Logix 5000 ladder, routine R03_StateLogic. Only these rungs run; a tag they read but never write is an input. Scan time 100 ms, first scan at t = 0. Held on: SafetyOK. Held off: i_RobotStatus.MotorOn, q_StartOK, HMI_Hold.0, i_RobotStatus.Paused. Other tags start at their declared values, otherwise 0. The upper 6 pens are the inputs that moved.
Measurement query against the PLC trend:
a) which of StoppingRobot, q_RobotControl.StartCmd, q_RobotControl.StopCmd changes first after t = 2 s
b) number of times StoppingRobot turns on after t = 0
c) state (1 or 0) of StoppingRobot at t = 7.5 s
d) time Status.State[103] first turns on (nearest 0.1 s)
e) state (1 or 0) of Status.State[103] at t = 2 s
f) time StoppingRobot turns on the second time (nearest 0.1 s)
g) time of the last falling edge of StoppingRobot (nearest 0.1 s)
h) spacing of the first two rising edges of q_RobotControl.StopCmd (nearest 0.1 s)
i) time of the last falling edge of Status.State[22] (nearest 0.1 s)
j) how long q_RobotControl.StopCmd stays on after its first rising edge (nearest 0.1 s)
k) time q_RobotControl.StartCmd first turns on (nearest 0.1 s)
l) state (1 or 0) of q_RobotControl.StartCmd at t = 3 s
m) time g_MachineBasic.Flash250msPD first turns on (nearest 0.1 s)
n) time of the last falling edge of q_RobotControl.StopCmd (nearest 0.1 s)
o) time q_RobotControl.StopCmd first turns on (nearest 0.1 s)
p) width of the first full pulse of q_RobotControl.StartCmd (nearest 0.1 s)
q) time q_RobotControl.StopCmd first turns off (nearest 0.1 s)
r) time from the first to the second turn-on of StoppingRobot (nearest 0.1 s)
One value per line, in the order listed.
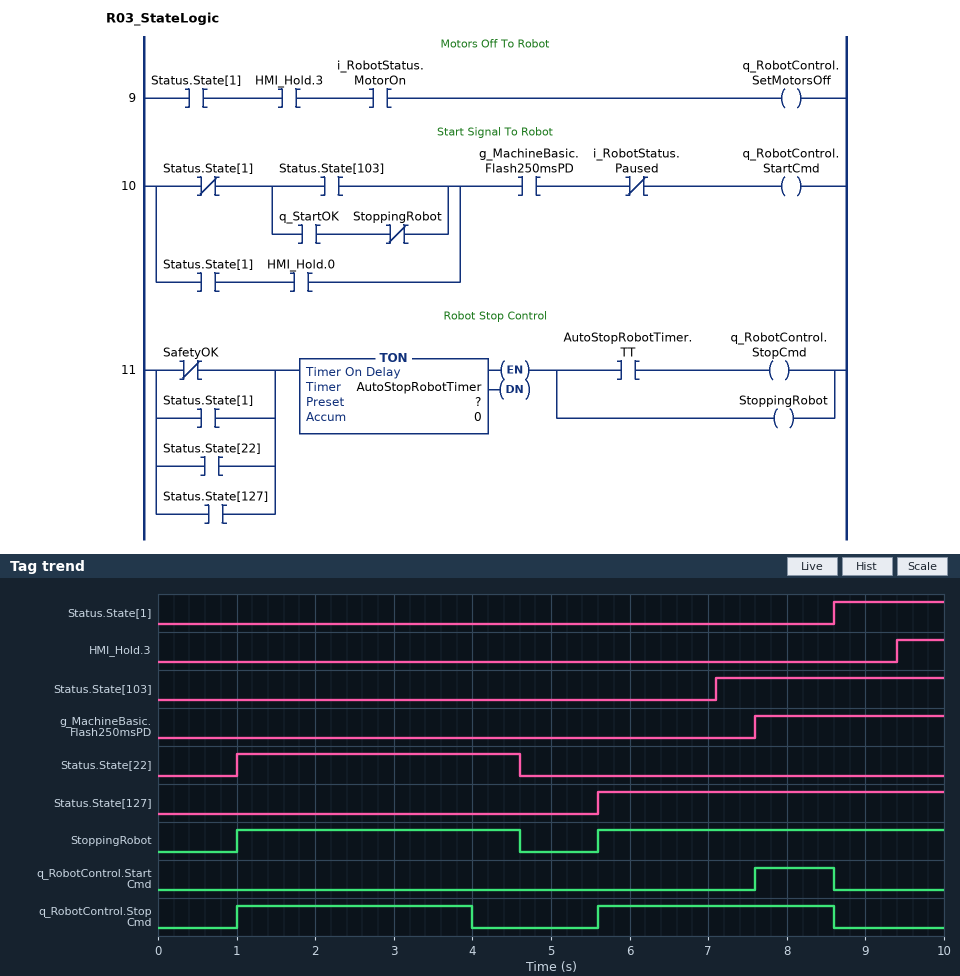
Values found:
q_RobotControl.StopCmd
2
1
7.1 s
0
5.6 s
4.6 s
4.6 s
4.6 s
3.0 s
7.6 s
0
7.6 s
8.6 s
1.0 s
1.0 s
4.0 s
4.6 s
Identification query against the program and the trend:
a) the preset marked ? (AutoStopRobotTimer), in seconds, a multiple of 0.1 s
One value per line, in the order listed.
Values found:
3.0 s
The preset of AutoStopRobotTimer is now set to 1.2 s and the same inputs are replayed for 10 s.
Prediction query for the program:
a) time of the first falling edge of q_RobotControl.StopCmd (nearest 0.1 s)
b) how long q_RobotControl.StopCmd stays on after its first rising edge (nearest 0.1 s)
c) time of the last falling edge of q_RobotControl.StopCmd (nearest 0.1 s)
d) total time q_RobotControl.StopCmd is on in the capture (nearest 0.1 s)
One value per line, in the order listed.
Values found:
2.2 s
1.2 s
6.8 s
2.4 s
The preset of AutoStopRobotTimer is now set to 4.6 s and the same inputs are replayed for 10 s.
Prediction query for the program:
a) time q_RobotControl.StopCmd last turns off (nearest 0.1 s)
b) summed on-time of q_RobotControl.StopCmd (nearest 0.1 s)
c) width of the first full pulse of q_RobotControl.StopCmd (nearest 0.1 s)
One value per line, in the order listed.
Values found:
4.6 s
8.0 s
3.6 s
